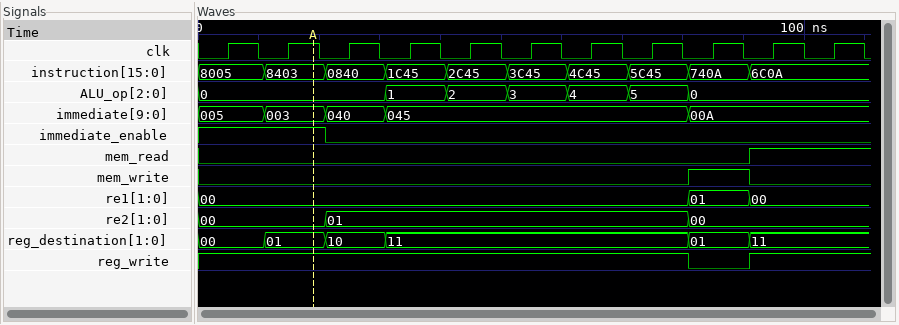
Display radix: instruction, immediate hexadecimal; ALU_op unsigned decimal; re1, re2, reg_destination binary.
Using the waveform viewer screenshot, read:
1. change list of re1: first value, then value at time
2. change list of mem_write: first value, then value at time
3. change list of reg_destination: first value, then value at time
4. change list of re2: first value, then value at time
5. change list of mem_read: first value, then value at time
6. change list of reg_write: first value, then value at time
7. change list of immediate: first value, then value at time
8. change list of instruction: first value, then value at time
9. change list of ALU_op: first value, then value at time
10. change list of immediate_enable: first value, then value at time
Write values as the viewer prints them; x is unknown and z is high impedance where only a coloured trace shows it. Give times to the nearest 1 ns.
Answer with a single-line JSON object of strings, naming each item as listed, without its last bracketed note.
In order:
{"change list of re1: first value, then value at time": "00, 01 at 81 ns, 00 at 91 ns", "change list of mem_write: first value, then value at time": "0, 1 at 81 ns, 0 at 91 ns", "change list of reg_destination: first value, then value at time": "00, 01 at 11 ns, 10 at 21 ns, 11 at 31 ns, 01 at 81 ns, 11 at 91 ns", "change list of re2: first value, then value at time": "00, 01 at 21 ns, 00 at 81 ns", "change list of mem_read: first value, then value at time": "0, 1 at 91 ns", "change list of reg_write: first value, then value at time": "1, 0 at 81 ns, 1 at 91 ns", "change list of immediate: first value, then value at time": "005, 003 at 11 ns, 040 at 21 ns, 045 at 31 ns, 00A at 81 ns", "change list of instruction: first value, then value at time": "8005, 8403 at 11 ns, 0840 at 21 ns, 1C45 at 31 ns, 2C45 at 41 ns, 3C45 at 51 ns, 4C45 at 61 ns, 5C45 at 71 ns, 740A at 81 ns, 6C0A at 91 ns", "change list of ALU_op: first value, then value at time": "0, 1 at 31 ns, 2 at 41 ns, 3 at 51 ns, 4 at 61 ns, 5 at 71 ns, 0 at 81 ns", "change list of immediate_enable: first value, then value at time": "1, 0 at 21 ns"}
